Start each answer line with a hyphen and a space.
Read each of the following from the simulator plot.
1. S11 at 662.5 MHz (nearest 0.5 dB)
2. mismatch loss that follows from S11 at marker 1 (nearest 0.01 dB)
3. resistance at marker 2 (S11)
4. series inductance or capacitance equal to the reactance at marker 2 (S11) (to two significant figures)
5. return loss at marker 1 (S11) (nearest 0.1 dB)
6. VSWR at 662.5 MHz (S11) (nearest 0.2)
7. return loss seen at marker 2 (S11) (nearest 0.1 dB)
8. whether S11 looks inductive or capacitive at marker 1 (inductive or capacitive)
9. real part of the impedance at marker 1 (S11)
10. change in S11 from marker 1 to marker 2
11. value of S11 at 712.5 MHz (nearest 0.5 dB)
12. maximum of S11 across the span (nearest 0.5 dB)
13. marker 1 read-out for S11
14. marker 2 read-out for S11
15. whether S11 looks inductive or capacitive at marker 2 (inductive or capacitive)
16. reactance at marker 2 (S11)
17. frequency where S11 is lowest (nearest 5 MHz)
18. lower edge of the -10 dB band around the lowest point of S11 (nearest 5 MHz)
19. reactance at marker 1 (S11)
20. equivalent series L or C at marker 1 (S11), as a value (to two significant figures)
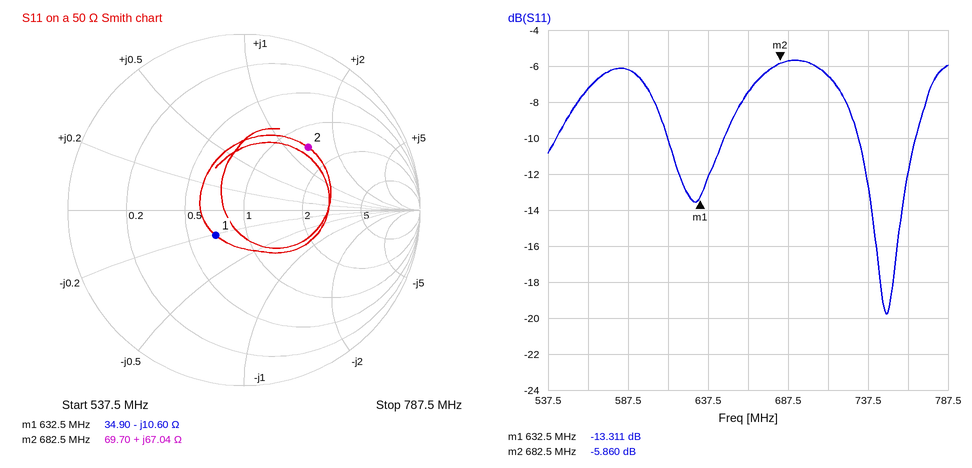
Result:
- -7.5 dB
- 0.21 dB
- 69.70 Ω
- 16 nH
- 13.3 dB
- 2.4
- 5.9 dB
- capacitive
- 34.90 Ω
- 7.451 dB
- -6.5 dB
- -5.5 dB
- -13.311 dB
- -5.860 dB
- inductive
- +67.04 Ω
- 750 MHz
- 730 MHz
- -10.60 Ω
- 24 pF
